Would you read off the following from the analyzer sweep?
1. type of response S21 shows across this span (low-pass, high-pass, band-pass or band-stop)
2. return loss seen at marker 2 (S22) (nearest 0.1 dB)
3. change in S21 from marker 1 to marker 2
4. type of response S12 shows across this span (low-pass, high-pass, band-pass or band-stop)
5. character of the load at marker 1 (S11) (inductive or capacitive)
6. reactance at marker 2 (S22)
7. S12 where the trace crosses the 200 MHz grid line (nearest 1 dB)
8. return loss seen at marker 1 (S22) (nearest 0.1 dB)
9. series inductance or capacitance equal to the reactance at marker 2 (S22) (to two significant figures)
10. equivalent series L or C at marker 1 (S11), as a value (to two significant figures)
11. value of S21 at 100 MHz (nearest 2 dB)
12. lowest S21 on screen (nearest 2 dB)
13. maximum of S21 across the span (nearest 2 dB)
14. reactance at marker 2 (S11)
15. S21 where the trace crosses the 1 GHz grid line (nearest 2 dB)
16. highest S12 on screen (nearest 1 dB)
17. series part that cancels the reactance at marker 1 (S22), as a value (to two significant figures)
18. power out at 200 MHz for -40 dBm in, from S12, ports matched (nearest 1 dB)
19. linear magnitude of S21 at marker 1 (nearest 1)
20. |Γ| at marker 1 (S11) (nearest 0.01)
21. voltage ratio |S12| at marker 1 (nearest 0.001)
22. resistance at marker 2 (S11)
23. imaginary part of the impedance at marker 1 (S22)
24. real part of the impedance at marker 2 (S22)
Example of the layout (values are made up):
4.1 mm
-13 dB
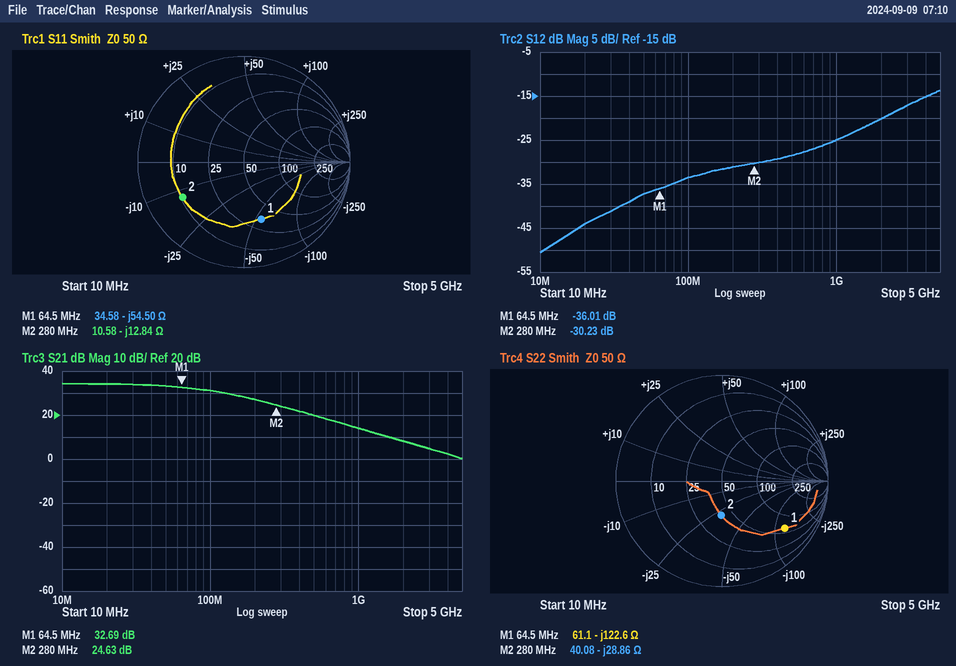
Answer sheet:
low-pass
9.8 dB
-8.06 dB
high-pass
capacitive
-28.86 Ω
-31 dB
2.6 dB
20 pF
45 pF
32 dB
0 dB
34 dB
-12.84 Ω
14 dB
-14 dB
300 nH
-71 dBm
43
0.56
0.016
10.58 Ω
-122.6 Ω
40.08 Ω
